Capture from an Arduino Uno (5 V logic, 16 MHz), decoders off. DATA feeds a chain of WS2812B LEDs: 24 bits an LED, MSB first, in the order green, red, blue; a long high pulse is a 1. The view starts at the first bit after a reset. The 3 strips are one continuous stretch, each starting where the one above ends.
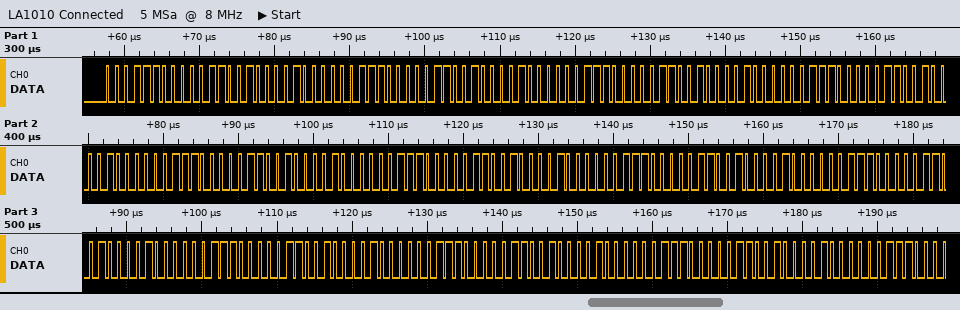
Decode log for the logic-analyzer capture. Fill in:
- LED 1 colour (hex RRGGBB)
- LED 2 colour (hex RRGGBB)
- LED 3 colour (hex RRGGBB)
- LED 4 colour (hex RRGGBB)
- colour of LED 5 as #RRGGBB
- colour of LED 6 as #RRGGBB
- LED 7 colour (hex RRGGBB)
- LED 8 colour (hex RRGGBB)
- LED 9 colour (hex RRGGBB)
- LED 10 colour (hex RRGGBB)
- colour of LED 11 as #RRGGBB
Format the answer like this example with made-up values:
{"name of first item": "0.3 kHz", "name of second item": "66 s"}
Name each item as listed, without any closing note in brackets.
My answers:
{"LED 1 colour": "#191C08", "LED 2 colour": "#191C08", "LED 3 colour": "#191C08", "LED 4 colour": "#191C08", "colour of LED 5 as #RRGGBB": "#191C08", "colour of LED 6 as #RRGGBB": "#191C08", "LED 7 colour": "#191C08", "LED 8 colour": "#191C08", "LED 9 colour": "#191C08", "LED 10 colour": "#191C08", "colour of LED 11 as #RRGGBB": "#191C08"}
